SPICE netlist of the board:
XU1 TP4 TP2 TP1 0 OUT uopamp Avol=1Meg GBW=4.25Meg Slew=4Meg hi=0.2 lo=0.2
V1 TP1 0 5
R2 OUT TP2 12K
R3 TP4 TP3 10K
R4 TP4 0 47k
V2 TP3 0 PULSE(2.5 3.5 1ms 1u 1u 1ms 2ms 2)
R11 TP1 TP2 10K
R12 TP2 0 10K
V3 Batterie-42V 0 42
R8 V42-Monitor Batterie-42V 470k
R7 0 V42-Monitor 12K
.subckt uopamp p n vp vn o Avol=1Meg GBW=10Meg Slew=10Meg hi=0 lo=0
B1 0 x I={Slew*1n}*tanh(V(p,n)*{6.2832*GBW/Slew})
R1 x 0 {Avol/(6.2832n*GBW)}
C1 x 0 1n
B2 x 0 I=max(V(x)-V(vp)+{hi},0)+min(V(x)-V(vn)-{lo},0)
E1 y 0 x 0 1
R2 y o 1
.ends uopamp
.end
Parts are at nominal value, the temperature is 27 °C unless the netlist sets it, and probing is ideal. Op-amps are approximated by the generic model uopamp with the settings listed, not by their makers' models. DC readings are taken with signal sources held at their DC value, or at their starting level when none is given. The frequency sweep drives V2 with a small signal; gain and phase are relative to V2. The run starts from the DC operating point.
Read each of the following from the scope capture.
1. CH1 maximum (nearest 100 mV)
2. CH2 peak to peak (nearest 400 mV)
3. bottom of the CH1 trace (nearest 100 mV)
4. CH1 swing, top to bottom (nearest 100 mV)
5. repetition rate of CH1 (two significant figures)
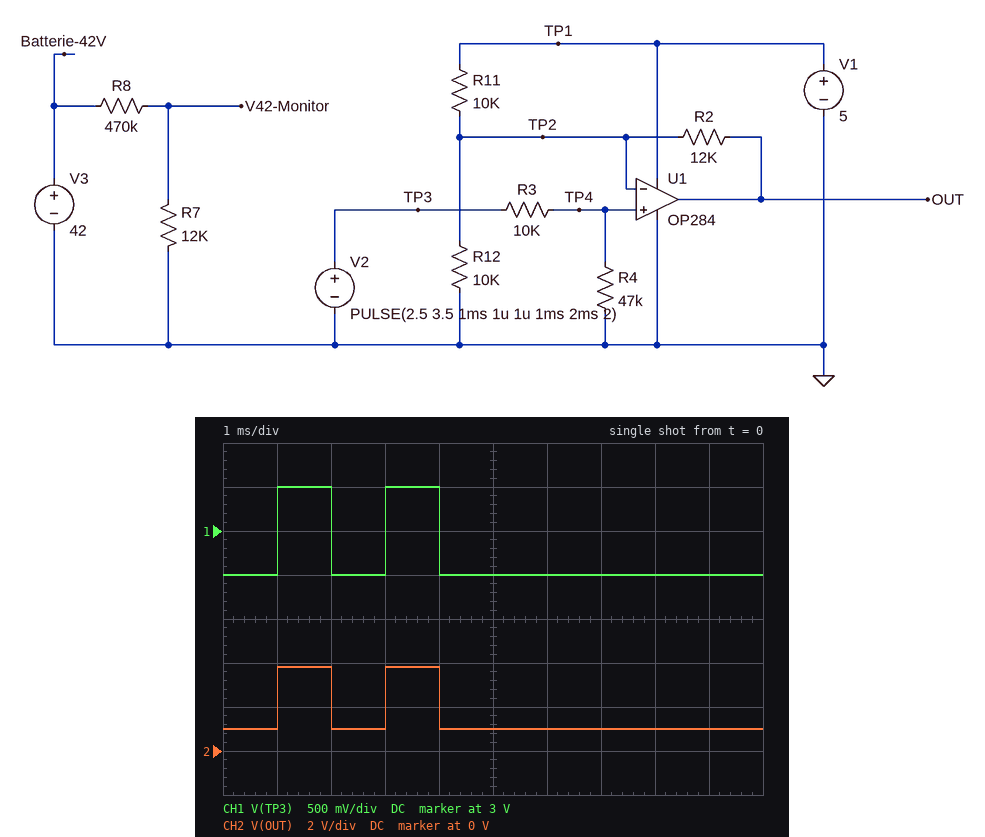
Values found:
3.5 V
2.8 V
2.5 V
1.0 V
500 Hz
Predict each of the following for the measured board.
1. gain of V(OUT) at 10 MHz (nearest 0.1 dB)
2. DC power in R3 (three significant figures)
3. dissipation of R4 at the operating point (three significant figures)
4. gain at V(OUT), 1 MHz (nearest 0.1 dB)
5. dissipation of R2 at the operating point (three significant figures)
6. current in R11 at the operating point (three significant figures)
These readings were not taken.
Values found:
-9.2 dB
19.2 µW
90.4 µW
6.8 dB
92.3 µW
294 µA
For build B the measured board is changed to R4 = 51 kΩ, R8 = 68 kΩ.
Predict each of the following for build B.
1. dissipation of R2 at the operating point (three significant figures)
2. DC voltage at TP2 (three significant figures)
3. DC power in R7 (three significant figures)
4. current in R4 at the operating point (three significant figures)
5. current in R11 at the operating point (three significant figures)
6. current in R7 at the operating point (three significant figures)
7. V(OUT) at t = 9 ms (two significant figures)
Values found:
80.6 µW
2.09 V
3.31 mW
41.0 µA
291 µA
525 µA
1.1 V
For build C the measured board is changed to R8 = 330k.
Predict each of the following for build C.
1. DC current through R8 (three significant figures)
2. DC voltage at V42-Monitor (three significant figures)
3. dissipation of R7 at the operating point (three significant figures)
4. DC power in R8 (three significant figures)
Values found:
123 µA
1.47 V
181 µW
4.98 mW
